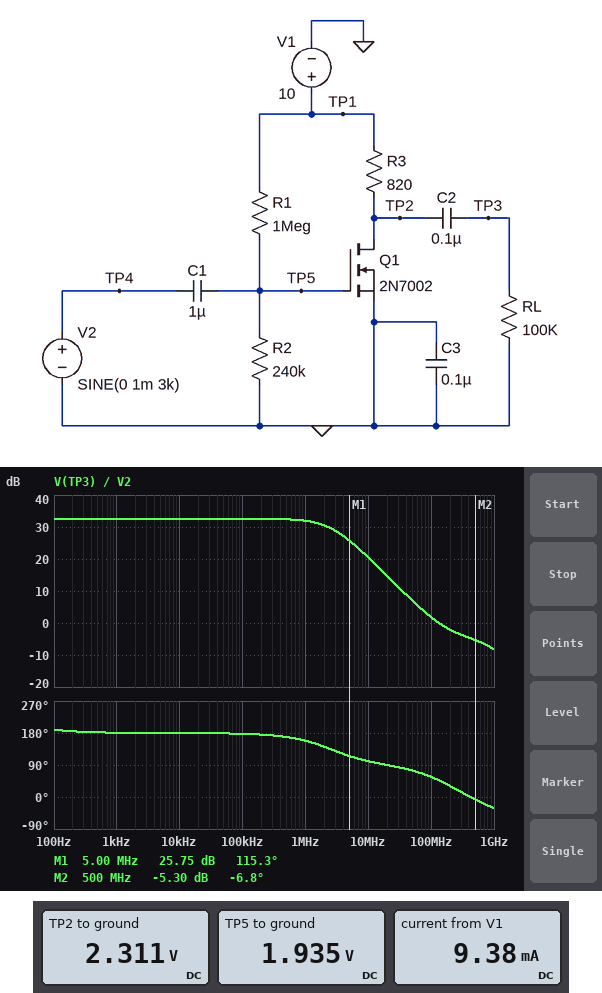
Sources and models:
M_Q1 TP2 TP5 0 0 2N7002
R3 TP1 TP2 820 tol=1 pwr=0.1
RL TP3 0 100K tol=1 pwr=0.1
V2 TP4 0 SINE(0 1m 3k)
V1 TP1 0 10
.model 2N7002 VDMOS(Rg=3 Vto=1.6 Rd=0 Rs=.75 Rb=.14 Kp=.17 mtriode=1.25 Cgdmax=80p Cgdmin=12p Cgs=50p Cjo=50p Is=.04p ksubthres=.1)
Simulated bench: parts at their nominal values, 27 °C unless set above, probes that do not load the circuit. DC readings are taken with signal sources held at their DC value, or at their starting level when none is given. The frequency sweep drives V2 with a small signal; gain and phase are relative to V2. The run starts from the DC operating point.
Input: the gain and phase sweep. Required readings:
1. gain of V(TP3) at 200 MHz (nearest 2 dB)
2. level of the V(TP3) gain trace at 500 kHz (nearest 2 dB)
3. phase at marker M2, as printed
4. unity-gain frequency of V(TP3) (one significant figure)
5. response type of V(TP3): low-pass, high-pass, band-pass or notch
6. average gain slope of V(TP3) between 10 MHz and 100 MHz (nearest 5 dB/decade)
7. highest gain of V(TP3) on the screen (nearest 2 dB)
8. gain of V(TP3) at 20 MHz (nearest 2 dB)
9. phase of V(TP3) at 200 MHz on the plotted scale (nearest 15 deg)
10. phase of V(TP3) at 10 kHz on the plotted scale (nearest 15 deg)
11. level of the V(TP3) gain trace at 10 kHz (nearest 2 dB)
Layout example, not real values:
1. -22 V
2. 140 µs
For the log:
1. -2 dB
2. 32 dB
3. -6.8 deg
4. 100 MHz
5. low-pass
6. -20 dB/decade
7. 32 dB
8. 14 dB
9. 30 deg
10. 180 deg
11. 32 dB
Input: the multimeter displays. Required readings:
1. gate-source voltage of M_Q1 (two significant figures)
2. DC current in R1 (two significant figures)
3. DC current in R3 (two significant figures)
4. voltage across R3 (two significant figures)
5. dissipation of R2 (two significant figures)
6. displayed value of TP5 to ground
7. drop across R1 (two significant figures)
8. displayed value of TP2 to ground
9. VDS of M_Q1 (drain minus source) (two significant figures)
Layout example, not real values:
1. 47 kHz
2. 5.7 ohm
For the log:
1. 1.9 V
2. 8.1 µA
3. 9.4 mA
4. 7.7 V
5. 16 µW
6. 1.935 V
7. 8.1 V
8. 2.311 V
9. 2.3 V
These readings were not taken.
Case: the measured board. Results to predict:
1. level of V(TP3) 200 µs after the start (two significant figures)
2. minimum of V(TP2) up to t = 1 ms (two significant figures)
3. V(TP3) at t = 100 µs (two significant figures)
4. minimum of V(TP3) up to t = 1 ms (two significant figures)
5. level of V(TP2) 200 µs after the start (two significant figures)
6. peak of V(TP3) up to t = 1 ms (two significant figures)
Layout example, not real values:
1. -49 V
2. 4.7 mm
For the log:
1. 25 mV
2. 2.3 V
3. -40 mV
4. -42 mV
5. 2.3 V
6. 43 mV
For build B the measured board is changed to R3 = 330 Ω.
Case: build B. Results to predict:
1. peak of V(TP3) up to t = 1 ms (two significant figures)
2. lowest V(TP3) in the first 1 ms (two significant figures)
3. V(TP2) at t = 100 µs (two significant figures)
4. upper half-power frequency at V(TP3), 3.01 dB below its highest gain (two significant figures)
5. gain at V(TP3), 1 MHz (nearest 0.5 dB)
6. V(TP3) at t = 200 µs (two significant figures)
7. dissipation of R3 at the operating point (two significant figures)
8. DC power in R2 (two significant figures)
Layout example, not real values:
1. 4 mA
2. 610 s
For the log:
1. 17 mV
2. -17 mV
3. 6.9 V
4. 13 MHz
5. 24.5 dB
6. 10 mV
7. 29 mW
8. 16 µW
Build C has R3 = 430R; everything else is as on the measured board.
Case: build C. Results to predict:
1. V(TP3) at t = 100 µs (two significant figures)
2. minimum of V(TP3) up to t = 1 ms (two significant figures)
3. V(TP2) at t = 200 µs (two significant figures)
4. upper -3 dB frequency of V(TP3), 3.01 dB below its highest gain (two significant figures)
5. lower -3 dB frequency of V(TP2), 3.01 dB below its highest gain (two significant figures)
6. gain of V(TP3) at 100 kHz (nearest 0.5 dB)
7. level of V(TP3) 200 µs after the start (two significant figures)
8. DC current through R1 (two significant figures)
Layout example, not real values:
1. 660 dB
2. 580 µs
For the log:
1. -21 mV
2. -22 mV
3. 6.0 V
4. 9.6 MHz
5. 820 mHz
6. 27.0 dB
7. 13 mV
8. 8.1 µA
